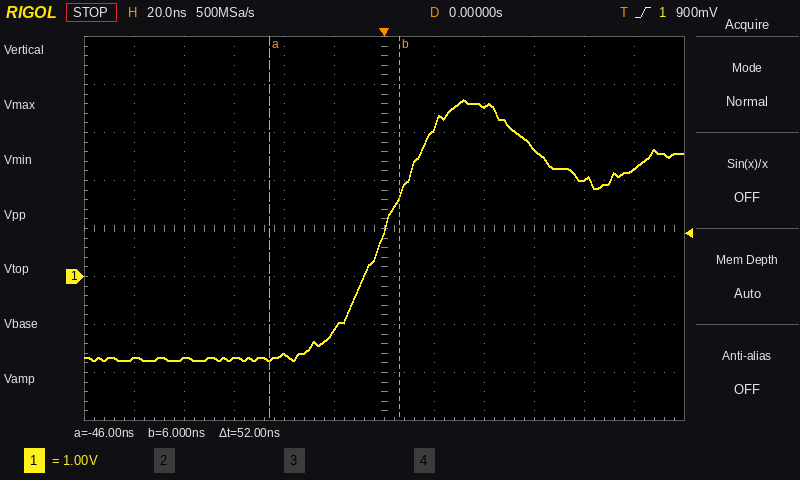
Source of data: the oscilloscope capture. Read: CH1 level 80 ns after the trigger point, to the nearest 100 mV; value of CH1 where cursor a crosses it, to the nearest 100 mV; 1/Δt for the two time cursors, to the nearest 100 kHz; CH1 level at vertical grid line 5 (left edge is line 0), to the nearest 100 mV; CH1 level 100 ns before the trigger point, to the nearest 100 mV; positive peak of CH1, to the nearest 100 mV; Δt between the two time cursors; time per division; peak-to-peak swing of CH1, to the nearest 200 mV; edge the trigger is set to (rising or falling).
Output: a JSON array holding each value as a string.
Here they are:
["2.0 V", "-1.7 V", "19.2 MHz", "-1.1 V", "-1.7 V", "3.7 V", "52 ns", "20 ns", "5.4 V", "rising"]
